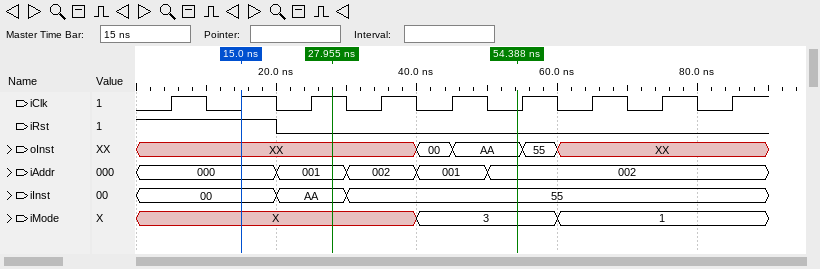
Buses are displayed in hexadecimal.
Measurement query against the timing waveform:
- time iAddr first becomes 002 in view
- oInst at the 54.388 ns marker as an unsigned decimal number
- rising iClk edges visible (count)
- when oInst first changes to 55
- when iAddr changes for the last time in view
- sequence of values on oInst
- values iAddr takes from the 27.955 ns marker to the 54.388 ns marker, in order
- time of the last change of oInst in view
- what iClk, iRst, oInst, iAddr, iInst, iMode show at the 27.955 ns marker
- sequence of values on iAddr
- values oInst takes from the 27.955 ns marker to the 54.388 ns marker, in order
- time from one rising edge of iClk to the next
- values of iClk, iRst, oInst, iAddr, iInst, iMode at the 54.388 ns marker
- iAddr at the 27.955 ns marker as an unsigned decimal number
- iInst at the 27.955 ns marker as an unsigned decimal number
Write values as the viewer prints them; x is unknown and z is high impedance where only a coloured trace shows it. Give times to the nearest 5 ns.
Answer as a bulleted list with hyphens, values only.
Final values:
- 30 ns
- 170
- 9
- 55 ns
- 50 ns
- XX, 00, AA, 55, XX
- 001, 002, 001, 002
- 60 ns
- iClk=1, iRst=0, oInst=XX, iAddr=001, iInst=AA, iMode=X
- 000, 001, 002, 001, 002
- XX, 00, AA
- 10 ns
- iClk=0, iRst=0, oInst=AA, iAddr=002, iInst=55, iMode=3
- 1
- 170
